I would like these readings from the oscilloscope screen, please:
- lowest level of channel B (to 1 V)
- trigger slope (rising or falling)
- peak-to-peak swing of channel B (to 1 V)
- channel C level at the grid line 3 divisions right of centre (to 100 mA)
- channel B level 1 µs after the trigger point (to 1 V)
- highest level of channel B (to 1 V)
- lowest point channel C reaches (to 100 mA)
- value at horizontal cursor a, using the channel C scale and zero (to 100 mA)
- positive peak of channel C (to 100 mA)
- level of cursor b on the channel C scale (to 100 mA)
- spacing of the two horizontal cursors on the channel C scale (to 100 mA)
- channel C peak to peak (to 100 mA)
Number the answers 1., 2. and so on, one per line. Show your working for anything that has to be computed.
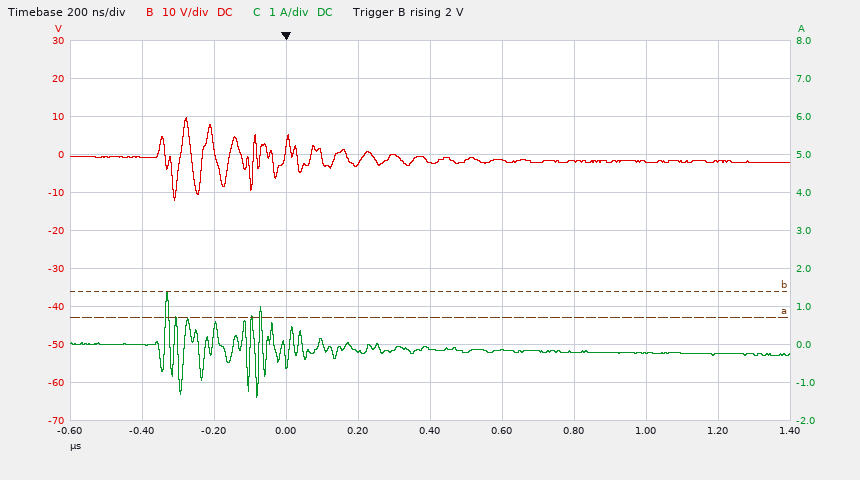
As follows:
1. -12 V
2. rising
3. 10 V − (-12 V) = 22 V
4. -200 mA
5. -2 V
6. 10 V
7. -1.4 A
8. 700 mA
9. 1.4 A
10. 1.4 A
11. 700 mA
12. 1.4 A − (-1.4 A) = 2.8 A
